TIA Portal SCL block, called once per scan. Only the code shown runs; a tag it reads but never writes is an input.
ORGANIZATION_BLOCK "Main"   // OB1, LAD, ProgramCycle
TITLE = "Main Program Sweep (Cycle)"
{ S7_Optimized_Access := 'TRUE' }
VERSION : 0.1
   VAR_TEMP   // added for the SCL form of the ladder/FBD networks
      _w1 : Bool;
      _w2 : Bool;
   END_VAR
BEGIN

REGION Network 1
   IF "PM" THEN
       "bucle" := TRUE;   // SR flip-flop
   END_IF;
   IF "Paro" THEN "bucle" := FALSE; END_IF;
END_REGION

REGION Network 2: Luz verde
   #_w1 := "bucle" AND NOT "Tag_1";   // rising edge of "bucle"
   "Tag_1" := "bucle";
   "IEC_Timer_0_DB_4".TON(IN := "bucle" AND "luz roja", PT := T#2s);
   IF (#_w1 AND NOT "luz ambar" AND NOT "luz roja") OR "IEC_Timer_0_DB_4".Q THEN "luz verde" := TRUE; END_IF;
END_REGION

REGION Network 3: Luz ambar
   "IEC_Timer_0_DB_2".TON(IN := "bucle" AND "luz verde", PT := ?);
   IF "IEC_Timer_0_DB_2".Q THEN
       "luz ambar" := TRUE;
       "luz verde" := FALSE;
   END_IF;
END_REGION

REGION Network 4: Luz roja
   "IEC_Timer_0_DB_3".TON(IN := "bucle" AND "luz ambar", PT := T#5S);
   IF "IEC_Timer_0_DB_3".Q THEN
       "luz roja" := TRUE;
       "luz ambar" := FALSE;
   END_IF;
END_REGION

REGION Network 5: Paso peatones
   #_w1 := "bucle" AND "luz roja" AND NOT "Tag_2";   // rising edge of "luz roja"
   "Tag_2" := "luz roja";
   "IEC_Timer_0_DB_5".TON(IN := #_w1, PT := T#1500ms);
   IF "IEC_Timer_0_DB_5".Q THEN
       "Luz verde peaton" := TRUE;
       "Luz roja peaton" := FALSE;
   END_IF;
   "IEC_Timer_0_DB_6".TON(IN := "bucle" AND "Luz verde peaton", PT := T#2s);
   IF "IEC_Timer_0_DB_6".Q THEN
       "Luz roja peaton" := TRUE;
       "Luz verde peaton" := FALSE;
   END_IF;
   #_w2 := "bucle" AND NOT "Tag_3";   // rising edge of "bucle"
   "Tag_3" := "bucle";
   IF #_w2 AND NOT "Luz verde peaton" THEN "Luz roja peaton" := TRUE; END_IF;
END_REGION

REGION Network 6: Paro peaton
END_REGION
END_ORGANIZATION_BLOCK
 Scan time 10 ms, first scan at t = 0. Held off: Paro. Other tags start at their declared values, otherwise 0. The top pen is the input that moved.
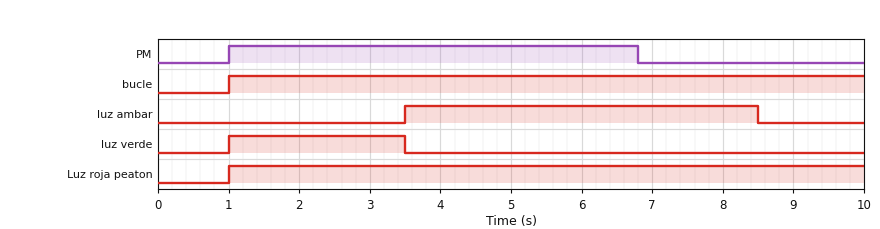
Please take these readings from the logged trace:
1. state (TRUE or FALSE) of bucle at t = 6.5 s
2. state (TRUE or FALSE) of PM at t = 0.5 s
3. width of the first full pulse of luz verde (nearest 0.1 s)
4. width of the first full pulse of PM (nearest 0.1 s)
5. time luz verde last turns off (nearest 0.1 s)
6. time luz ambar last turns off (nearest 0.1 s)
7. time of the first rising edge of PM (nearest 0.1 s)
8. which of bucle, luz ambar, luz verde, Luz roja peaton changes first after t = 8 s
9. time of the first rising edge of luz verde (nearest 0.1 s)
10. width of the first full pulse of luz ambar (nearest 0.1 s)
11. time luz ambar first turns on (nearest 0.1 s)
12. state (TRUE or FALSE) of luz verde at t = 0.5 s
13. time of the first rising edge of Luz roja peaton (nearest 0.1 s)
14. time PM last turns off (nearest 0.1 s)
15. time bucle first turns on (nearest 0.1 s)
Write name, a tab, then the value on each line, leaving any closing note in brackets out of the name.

state (TRUE or FALSE) of bucle at t = 6.5 s	TRUE
state (TRUE or FALSE) of PM at t = 0.5 s	FALSE
width of the first full pulse of luz verde	2.5 s
width of the first full pulse of PM	5.8 s
time luz verde last turns off	3.5 s
time luz ambar last turns off	8.5 s
time of the first rising edge of PM	1.0 s
which of bucle, luz ambar, luz verde, Luz roja peaton changes first after t = 8 s	luz ambar
time of the first rising edge of luz verde	1.0 s
width of the first full pulse of luz ambar	5.0 s
time luz ambar first turns on	3.5 s
state (TRUE or FALSE) of luz verde at t = 0.5 s	FALSE
time of the first rising edge of Luz roja peaton	1.0 s
time PM last turns off	6.8 s
time bucle first turns on	1.0 s
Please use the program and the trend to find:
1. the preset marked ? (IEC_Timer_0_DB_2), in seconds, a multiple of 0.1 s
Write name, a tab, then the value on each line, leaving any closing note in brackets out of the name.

the preset marked ? (IEC_Timer_0_DB_2), in seconds, a multiple of 0.1 s	2.5 s
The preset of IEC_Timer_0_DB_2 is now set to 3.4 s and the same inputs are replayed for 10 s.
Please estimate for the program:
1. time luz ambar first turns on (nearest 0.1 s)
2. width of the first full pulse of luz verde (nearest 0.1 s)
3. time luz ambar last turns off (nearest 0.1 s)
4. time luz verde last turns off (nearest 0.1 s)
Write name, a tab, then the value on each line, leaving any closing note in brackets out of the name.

time luz ambar first turns on	4.4 s
width of the first full pulse of luz verde	3.4 s
time luz ambar last turns off	9.4 s
time luz verde last turns off	4.4 s
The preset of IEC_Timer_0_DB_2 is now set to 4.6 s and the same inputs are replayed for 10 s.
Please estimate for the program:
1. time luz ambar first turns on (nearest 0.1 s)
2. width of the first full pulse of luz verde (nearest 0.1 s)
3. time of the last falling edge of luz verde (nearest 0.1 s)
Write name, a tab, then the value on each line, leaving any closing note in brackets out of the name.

time luz ambar first turns on	5.6 s
width of the first full pulse of luz verde	4.6 s
time of the last falling edge of luz verde	5.6 s
